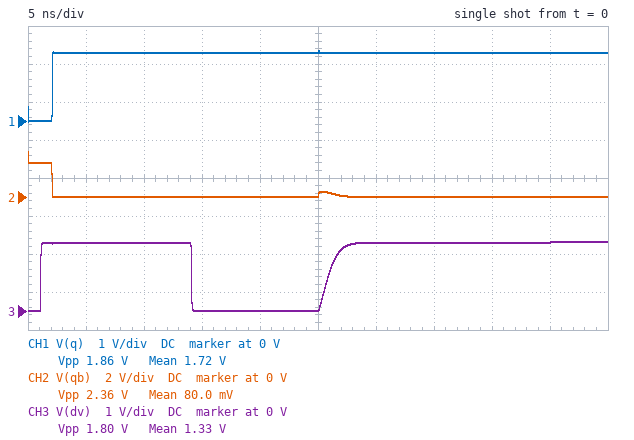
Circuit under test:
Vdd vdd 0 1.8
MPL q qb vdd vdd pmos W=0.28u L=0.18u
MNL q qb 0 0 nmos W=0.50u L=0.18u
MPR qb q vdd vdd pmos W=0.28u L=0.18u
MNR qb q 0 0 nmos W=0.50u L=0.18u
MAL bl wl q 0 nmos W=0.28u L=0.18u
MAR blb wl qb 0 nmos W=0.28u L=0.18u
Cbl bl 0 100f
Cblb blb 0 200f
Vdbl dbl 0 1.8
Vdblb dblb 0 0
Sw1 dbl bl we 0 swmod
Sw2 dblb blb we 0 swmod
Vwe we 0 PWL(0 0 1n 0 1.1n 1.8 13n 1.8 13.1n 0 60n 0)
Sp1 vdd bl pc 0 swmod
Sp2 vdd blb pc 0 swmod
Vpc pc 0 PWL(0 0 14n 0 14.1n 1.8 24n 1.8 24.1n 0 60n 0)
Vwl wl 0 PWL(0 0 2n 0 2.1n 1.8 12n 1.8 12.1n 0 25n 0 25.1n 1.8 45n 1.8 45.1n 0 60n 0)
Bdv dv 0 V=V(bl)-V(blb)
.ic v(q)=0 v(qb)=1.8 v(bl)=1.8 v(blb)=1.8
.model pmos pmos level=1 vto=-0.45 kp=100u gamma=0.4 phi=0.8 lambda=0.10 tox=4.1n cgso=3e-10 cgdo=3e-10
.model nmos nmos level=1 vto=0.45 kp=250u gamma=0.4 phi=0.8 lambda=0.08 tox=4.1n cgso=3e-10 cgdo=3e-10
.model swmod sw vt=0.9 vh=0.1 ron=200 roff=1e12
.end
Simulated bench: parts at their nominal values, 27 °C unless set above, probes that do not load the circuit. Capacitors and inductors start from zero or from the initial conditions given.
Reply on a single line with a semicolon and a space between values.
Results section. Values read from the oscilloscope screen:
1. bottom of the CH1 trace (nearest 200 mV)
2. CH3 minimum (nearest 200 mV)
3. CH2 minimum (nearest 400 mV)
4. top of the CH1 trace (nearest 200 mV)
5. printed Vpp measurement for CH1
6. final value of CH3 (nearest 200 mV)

0 V; 0 V; 0 V; 1.8 V; 1.86 V; 1.8 V
